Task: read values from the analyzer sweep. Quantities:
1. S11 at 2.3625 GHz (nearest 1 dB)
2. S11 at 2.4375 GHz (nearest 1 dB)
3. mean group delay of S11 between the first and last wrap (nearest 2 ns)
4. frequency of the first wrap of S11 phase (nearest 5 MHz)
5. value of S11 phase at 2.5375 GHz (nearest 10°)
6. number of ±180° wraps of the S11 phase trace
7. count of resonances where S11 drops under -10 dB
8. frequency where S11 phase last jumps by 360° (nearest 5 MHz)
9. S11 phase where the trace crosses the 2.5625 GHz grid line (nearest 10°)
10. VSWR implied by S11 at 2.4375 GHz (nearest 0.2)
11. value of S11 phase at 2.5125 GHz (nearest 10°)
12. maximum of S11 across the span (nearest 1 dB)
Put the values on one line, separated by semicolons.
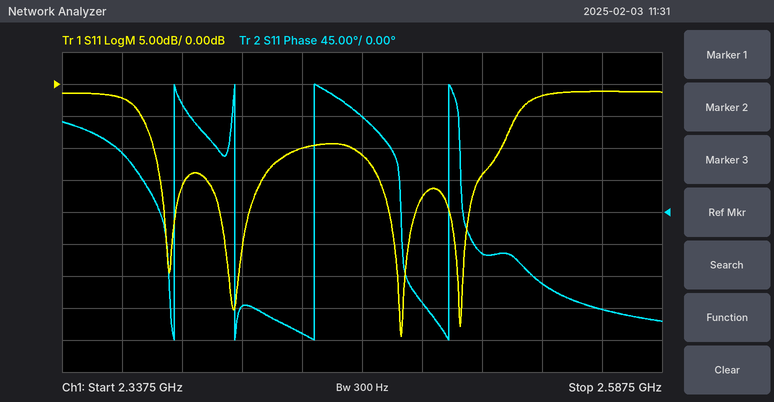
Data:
-2 dB; -10 dB; 26 ns; 2.385 GHz; -100°; 4; 4; 2.500 GHz; -140°; 2.0; -60°; -1 dB
